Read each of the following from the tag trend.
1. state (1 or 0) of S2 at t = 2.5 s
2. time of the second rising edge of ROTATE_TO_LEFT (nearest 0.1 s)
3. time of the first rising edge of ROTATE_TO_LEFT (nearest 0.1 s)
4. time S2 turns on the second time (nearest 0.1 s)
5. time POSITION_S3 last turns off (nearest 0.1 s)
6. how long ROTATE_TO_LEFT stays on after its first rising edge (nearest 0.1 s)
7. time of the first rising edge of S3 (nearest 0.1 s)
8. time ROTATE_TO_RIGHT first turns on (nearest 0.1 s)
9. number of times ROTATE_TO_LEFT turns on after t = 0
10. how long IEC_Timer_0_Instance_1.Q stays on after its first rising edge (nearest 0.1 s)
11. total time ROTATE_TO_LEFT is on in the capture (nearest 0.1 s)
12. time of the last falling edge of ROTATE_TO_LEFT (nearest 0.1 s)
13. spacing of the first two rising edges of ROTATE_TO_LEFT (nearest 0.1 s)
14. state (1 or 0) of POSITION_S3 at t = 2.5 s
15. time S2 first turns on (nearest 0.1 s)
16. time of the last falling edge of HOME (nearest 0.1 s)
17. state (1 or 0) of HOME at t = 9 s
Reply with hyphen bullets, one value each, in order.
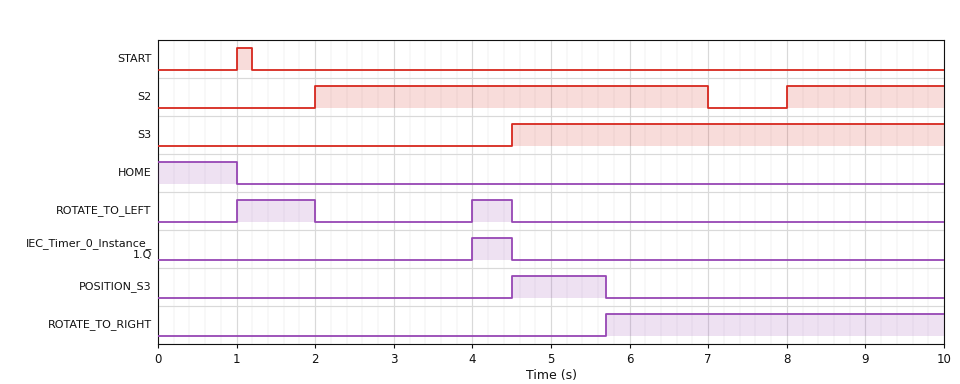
- 1
- 4.0 s
- 1.0 s
- 8.0 s
- 5.7 s
- 1.0 s
- 4.5 s
- 5.7 s
- 2
- 0.5 s
- 1.5 s
- 4.5 s
- 3.0 s
- 0
- 2.0 s
- 1.0 s
- 0
